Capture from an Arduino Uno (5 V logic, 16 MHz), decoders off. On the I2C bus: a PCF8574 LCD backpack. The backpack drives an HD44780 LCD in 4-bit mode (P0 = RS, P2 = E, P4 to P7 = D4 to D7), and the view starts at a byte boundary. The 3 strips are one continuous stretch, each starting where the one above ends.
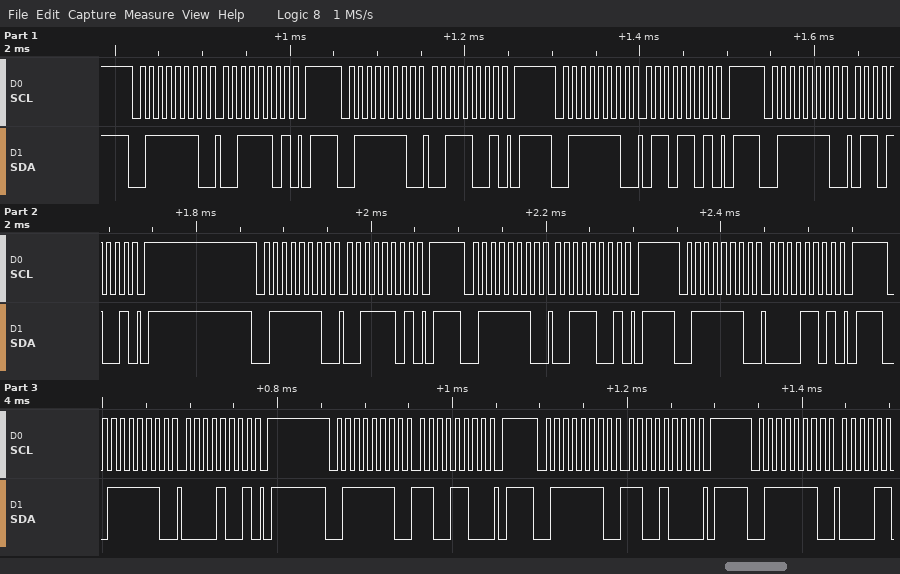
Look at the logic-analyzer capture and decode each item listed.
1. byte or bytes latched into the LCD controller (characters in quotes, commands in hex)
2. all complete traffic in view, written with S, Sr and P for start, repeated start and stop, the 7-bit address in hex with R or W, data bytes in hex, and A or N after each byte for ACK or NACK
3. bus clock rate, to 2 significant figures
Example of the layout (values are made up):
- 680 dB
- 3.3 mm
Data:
- '6' '0'
- S 3FW A 3D A P S 3FW A 39 A P S 3FW A 6D A P S 3FW A 69 A P S 3FW A 3D A P S 3FW A 39 A P S 3FW A 0D A P S 3FW A 09 A P S 3FW A CC A P S 3FW A C8 A P S 3FW A
- 100 kHz
